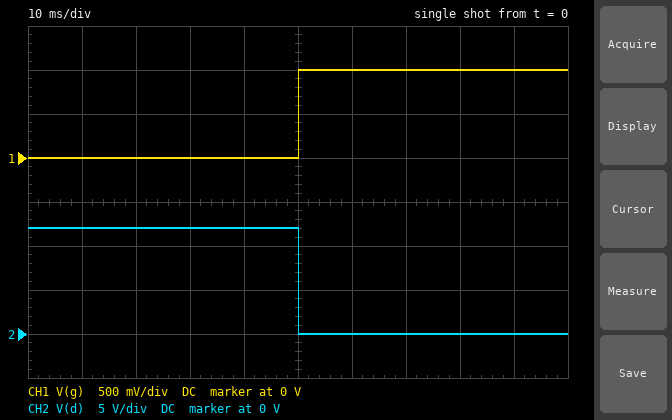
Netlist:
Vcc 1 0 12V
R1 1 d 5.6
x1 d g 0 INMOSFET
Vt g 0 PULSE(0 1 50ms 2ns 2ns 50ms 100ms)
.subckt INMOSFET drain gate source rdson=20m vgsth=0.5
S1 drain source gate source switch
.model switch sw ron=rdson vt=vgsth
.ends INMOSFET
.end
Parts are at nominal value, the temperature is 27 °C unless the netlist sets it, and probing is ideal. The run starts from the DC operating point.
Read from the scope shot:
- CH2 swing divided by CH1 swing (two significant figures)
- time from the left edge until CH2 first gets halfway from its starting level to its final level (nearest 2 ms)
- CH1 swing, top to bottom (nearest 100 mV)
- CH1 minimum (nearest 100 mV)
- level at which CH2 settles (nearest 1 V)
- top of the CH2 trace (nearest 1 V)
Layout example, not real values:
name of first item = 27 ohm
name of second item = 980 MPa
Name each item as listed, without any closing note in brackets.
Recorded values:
CH2 swing divided by CH1 swing = 12
time from the left edge until CH2 first gets halfway from its starting level to its final level = 50 ms
CH1 swing, top to bottom = 1.0 V
CH1 minimum = 0 V
level at which CH2 settles = 0 V
top of the CH2 trace = 12 V
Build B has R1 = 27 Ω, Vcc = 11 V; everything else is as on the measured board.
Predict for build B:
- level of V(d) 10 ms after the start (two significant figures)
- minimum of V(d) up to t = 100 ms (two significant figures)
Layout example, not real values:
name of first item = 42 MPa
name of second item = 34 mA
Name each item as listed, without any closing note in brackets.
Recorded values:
level of V(d) 10 ms after the start = 11 V
minimum of V(d) up to t = 100 ms = 8.1 mV
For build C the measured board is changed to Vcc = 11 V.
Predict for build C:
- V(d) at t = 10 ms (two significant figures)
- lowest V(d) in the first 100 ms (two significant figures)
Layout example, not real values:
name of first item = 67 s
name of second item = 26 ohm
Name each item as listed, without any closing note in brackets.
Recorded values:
V(d) at t = 10 ms = 11 V
lowest V(d) in the first 100 ms = 39 mV
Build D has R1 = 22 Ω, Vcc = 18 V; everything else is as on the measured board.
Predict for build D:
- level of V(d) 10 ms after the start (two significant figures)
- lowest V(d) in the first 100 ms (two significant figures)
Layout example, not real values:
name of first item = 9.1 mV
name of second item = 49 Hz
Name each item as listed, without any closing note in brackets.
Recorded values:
level of V(d) 10 ms after the start = 18 V
lowest V(d) in the first 100 ms = 16 mV
